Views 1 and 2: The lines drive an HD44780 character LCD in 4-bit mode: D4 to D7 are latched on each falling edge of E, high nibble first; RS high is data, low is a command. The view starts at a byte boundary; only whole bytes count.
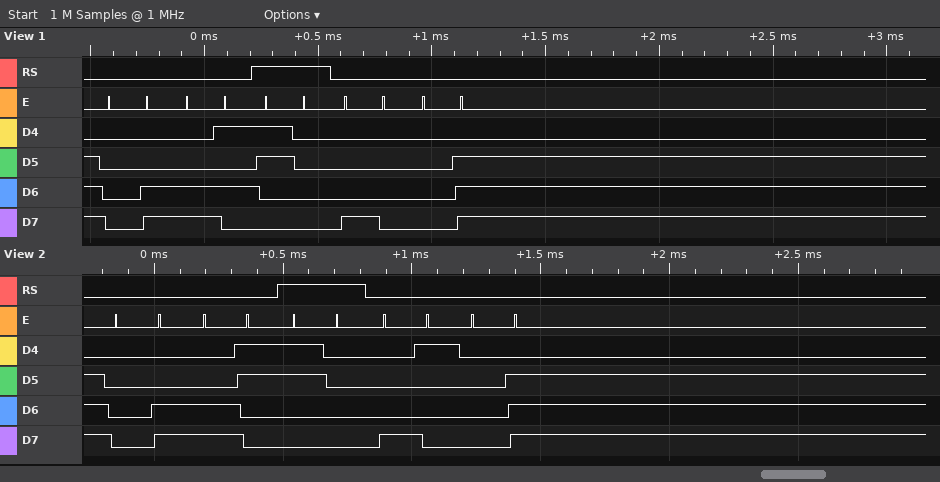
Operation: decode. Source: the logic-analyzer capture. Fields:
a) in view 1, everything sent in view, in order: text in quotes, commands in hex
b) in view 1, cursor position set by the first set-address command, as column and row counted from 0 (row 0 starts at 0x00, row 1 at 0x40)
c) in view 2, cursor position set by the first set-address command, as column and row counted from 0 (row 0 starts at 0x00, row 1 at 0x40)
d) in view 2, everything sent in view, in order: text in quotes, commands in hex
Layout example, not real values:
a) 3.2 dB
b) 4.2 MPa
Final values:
a) 0x0C 0xC5 "0" 0x80 0x0E
b) column 5, row 1
c) column 3, row 1
d) 0x0C 0xC3 "0" 0x81 0x0E
